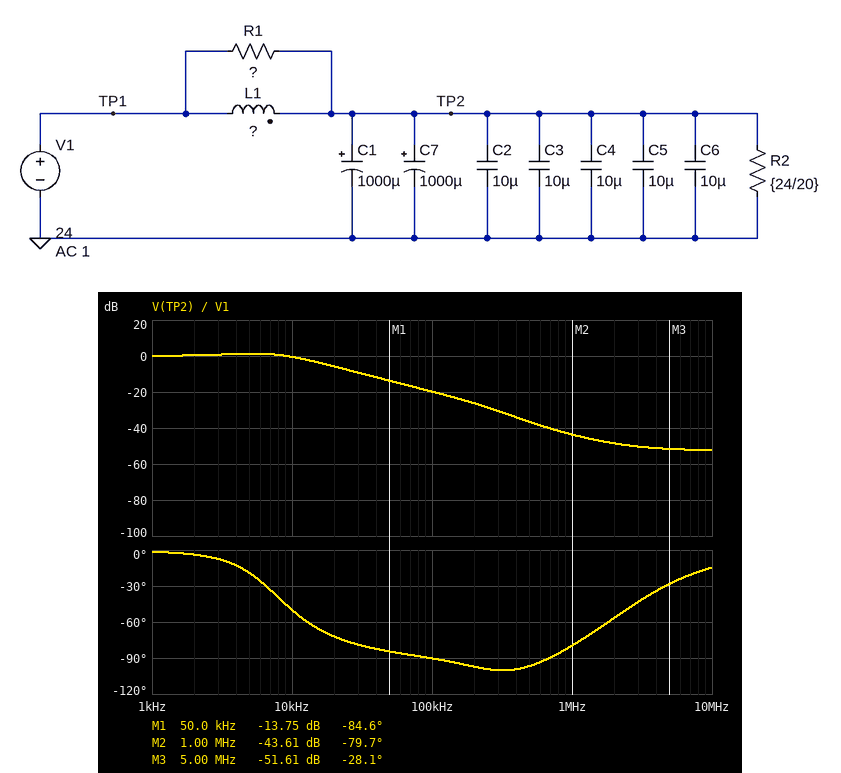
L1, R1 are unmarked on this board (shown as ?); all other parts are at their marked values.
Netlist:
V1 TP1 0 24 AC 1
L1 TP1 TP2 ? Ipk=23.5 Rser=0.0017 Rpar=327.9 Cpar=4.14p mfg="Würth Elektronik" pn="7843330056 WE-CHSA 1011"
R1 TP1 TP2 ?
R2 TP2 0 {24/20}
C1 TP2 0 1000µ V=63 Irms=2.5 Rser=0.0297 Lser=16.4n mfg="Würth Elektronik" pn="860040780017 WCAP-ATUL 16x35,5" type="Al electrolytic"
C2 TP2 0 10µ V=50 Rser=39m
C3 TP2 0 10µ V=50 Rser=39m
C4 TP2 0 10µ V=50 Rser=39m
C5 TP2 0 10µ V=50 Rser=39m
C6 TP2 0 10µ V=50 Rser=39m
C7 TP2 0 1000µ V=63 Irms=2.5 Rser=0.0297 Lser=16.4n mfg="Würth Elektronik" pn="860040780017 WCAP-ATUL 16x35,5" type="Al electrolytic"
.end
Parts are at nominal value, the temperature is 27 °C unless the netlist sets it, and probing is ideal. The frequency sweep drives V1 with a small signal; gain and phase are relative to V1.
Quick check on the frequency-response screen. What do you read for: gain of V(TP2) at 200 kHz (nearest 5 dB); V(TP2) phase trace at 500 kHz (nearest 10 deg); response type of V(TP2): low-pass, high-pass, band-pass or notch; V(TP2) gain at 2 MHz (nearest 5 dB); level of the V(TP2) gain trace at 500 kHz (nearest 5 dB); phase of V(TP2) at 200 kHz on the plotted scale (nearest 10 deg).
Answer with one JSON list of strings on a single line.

["-25 dB", "-100 deg", "low-pass", "-50 dB", "-35 dB", "-100 deg"]
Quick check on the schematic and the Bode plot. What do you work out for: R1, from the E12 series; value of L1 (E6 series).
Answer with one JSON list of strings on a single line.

["3.3 Ω", "220 nH"]
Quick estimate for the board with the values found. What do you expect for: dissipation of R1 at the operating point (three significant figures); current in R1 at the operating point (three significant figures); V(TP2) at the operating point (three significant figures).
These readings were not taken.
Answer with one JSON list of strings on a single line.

["349 µW", "10.3 mA", "24.0 V"]
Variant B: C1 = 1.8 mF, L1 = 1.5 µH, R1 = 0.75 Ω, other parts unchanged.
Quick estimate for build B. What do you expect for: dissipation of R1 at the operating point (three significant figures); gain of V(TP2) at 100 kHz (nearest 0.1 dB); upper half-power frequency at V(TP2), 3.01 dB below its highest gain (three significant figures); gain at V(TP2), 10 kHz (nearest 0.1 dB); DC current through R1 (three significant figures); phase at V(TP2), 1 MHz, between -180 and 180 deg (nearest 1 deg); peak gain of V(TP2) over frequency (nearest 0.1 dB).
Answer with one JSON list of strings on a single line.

["1.53 mW", "-32.5 dB", "3.08 kHz", "-15.3 dB", "45.2 mA", "-17 deg", "4.1 dB"]
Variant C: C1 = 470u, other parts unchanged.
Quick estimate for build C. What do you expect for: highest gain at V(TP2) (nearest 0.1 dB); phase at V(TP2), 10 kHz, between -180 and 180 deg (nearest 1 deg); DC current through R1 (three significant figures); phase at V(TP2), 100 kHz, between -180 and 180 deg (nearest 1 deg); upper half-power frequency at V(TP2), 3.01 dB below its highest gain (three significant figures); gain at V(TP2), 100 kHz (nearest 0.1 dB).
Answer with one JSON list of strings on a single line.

["1.7 dB", "-47 deg", "10.3 mA", "-92 deg", "13.7 kHz", "-19.9 dB"]
